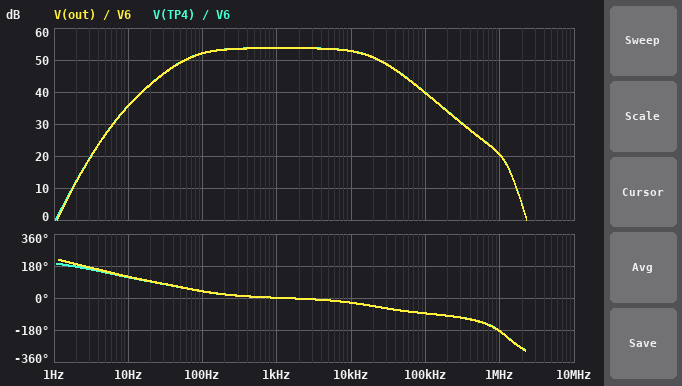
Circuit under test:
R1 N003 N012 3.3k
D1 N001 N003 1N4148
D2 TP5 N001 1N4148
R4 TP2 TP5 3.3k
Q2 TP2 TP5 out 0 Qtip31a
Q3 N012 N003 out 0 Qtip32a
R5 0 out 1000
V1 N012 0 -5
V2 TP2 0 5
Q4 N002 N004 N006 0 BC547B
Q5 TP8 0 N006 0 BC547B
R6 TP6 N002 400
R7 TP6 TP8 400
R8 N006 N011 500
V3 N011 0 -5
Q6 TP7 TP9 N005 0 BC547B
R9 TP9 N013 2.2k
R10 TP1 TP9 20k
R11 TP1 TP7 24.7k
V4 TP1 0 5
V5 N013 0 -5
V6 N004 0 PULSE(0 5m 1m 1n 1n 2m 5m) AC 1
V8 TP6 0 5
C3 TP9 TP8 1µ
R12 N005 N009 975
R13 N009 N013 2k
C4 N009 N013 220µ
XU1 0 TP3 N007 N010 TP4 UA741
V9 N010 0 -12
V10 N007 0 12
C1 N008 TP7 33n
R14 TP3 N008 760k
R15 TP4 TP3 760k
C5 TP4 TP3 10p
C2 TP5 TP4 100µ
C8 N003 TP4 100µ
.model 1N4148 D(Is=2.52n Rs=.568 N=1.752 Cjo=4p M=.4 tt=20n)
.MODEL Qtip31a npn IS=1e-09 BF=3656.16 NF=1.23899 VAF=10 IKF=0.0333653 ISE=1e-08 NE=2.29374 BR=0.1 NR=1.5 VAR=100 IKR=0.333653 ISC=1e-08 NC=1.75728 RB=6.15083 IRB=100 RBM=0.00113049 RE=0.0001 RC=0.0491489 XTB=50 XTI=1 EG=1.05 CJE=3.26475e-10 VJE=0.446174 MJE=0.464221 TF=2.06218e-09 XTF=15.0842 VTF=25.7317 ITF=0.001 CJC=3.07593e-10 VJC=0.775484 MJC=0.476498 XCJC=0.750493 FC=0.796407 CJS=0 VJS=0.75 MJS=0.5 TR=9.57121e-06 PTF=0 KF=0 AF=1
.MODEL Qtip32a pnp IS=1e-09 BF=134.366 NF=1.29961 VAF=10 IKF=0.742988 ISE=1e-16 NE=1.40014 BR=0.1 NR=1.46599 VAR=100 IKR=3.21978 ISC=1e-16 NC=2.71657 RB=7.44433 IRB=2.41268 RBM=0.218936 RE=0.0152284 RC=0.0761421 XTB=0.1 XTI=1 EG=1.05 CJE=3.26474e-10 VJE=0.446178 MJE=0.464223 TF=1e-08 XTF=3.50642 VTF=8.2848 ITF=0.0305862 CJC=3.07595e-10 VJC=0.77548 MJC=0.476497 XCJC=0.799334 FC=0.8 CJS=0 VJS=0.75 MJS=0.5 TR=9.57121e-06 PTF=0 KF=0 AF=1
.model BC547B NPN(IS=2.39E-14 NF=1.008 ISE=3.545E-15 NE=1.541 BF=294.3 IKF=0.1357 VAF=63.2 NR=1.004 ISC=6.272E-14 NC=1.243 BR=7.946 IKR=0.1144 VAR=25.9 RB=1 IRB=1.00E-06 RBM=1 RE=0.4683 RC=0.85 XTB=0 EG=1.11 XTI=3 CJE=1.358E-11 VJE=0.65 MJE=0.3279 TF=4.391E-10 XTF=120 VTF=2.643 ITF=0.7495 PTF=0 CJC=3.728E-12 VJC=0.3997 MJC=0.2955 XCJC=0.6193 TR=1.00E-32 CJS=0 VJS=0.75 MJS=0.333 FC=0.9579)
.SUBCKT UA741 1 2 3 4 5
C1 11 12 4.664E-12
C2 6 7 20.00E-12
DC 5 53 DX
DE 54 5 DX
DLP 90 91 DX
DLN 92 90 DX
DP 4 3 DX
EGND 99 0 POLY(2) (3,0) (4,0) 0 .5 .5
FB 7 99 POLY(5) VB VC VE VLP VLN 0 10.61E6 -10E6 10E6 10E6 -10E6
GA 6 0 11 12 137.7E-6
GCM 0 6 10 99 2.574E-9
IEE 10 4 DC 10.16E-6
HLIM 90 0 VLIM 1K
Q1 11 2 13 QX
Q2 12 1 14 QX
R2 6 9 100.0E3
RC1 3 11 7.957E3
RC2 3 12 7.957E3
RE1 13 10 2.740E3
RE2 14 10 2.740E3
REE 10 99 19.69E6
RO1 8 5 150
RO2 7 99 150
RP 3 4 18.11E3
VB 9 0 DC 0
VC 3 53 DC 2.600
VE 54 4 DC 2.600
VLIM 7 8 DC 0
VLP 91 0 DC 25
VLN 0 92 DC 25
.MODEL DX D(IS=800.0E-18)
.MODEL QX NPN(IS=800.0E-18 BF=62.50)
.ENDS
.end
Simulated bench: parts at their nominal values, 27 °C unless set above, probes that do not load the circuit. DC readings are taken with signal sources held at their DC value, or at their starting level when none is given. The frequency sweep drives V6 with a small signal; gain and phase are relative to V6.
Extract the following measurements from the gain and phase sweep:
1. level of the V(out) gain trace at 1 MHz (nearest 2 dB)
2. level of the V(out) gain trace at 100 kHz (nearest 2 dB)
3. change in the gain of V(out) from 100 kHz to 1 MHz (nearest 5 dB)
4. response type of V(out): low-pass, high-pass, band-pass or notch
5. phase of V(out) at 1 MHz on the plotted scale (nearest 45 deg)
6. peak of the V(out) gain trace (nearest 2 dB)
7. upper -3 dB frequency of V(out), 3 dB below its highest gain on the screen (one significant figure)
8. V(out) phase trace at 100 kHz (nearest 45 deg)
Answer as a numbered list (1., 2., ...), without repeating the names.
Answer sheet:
1. 20 dB
2. 40 dB
3. -20 dB
4. band-pass
5. -180 deg
6. 54 dB
7. 20 kHz
8. -90 deg
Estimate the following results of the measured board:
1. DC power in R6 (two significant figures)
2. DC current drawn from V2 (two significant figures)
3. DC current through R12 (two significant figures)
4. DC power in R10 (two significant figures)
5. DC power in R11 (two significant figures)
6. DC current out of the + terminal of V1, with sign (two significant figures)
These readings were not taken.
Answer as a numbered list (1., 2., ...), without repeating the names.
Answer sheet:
1. 7.4 mW
2. 56 mA
3. 140 µA
4. 4.1 mW
5. 460 µW
6. -56 mA
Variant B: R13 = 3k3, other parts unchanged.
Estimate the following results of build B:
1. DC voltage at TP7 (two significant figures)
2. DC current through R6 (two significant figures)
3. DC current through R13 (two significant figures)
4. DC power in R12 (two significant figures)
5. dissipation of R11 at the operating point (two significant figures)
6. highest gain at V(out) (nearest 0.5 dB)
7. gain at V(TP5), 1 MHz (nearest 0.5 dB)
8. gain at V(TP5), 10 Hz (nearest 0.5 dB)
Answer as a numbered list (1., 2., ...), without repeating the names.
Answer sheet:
1. 2.6 V
2. 4.3 mA
3. 97 µA
4. 9.2 µW
5. 230 µW
6. 53.0 dB
7. 20.0 dB
8. 35.0 dB
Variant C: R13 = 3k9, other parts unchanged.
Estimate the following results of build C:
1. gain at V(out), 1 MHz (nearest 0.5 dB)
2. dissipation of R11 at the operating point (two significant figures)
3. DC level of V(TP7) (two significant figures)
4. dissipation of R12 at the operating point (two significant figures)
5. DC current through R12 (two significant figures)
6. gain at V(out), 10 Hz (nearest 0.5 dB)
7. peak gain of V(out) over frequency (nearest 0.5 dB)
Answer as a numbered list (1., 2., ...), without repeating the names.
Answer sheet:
1. 19.5 dB
2. 180 µW
3. 2.9 V
4. 7.2 µW
5. 86 µA
6. 35.0 dB
7. 53.0 dB
